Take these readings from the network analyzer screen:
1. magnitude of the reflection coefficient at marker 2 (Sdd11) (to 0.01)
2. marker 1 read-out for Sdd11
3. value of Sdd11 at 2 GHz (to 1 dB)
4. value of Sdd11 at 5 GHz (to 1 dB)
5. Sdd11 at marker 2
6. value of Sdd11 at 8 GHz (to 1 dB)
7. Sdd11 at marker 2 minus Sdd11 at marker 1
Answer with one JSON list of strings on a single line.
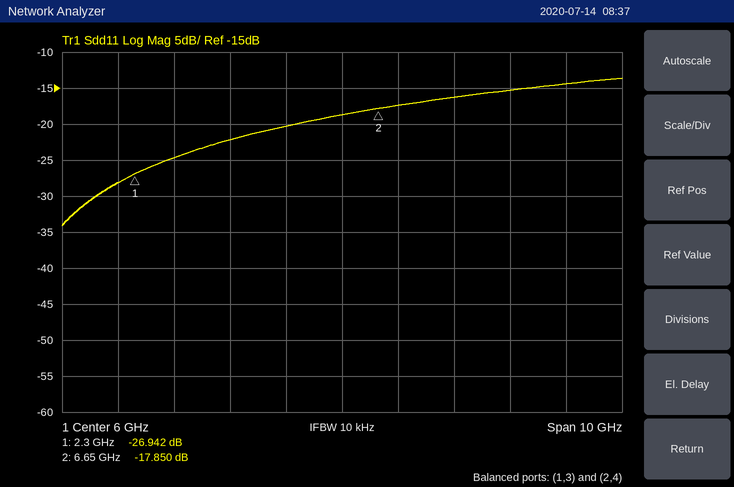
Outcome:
["0.13", "-26.942 dB", "-28 dB", "-20 dB", "-17.850 dB", "-16 dB", "9.092 dB"]
